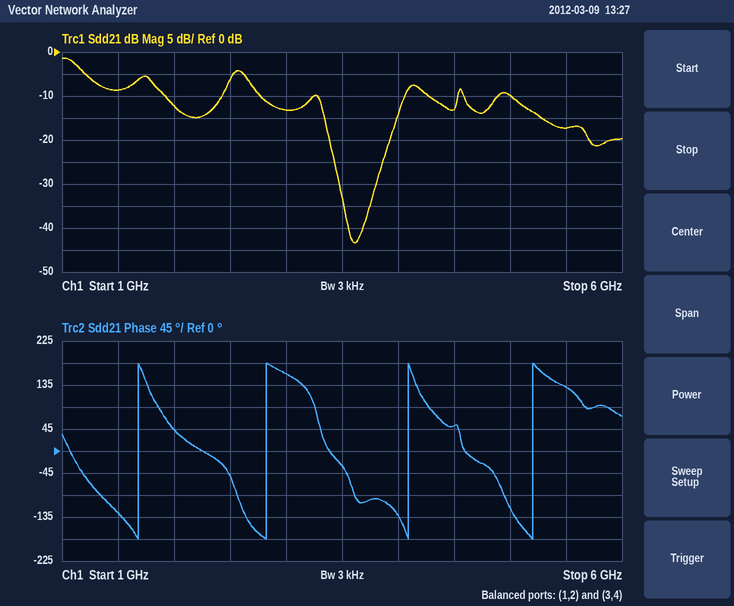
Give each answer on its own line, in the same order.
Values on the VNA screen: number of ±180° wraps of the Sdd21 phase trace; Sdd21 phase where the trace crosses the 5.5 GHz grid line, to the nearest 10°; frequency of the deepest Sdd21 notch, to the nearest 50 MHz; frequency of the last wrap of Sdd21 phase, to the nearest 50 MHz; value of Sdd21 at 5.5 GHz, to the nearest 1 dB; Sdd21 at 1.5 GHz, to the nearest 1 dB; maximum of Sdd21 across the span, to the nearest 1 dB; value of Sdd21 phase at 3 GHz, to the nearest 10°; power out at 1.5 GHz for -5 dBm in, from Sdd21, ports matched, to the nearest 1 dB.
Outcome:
4
130°
3.60 GHz
5.20 GHz
-17 dB
-9 dB
-1 dB
160°
-14 dBm
